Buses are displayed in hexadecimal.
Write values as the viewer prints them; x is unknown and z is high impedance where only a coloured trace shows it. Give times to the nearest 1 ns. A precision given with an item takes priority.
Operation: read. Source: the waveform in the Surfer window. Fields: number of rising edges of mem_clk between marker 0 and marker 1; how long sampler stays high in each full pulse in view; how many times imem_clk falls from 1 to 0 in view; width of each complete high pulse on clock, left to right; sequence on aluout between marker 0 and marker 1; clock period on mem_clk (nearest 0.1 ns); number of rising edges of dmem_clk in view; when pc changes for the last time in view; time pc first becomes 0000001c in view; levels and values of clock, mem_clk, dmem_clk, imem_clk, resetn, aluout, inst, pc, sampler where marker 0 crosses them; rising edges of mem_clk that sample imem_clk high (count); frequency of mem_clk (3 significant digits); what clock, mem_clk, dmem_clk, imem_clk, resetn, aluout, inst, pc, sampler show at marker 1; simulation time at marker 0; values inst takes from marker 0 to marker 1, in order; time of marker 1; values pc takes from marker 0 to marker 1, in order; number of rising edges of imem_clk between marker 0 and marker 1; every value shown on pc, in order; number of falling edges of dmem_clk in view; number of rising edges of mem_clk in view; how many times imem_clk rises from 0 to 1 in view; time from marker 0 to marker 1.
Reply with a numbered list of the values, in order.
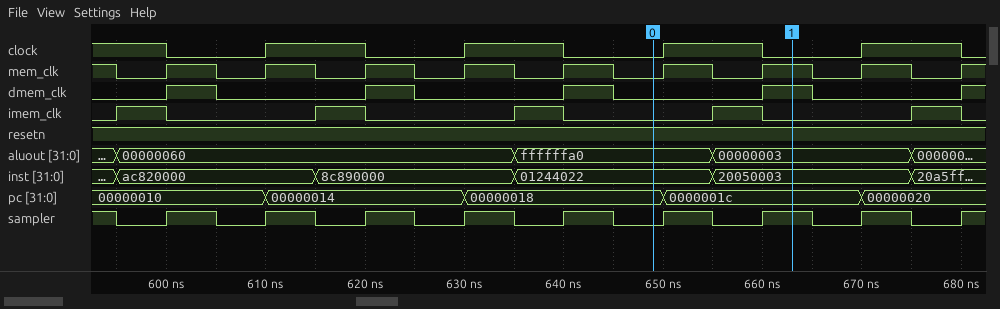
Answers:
1. 2
2. 5 ns, 5 ns, 5 ns, 5 ns, 5 ns, 5 ns, 5 ns, 5 ns
3. 5
4. 10 ns, 10 ns, 10 ns, 10 ns
5. ffffffa0, 00000003
6. 10 ns
7. 5
8. 670 ns
9. 650 ns
10. clock=0, mem_clk=0, dmem_clk=0, imem_clk=0, resetn=1, aluout=ffffffa0, inst=01244022, pc=00000018, sampler=0
11. 5
12. 100 MHz
13. clock=0, mem_clk=1, dmem_clk=1, imem_clk=0, resetn=1, aluout=00000003, inst=20050003, pc=0000001c, sampler=1
14. 649 ns
15. 01244022, 20050003
16. 663 ns
17. 00000018, 0000001c
18. 1
19. 00000010, 00000014, 00000018, 0000001c, 00000020
20. 4
21. 9
22. 5
23. 14 ns
